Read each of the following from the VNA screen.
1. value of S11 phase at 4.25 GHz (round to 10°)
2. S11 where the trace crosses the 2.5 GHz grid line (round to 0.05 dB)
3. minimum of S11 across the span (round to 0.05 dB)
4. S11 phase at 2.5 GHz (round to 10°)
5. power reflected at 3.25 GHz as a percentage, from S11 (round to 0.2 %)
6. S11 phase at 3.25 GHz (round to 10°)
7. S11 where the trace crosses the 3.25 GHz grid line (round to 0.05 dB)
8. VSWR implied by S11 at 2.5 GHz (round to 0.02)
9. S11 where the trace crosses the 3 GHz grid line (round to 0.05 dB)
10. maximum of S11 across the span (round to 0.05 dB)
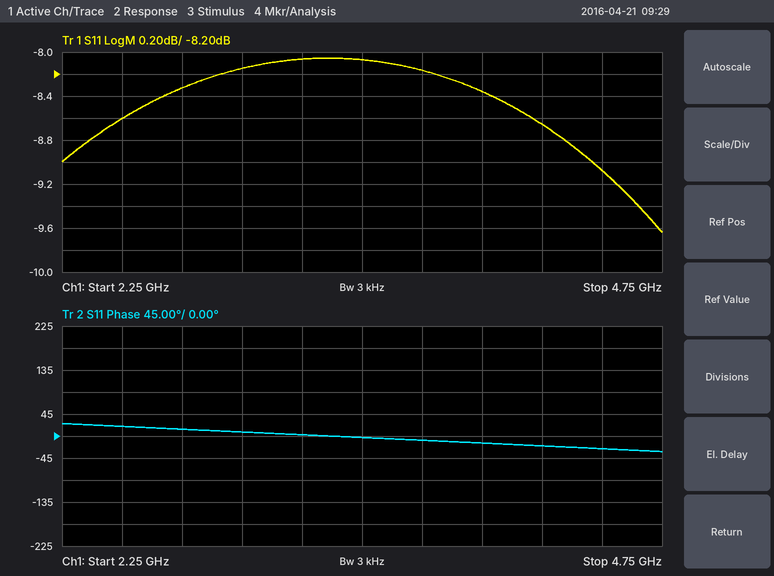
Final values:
-20°
-8.60 dB
-9.65 dB
20°
15.6 %
0°
-8.05 dB
2.18
-8.15 dB
-8.05 dB
